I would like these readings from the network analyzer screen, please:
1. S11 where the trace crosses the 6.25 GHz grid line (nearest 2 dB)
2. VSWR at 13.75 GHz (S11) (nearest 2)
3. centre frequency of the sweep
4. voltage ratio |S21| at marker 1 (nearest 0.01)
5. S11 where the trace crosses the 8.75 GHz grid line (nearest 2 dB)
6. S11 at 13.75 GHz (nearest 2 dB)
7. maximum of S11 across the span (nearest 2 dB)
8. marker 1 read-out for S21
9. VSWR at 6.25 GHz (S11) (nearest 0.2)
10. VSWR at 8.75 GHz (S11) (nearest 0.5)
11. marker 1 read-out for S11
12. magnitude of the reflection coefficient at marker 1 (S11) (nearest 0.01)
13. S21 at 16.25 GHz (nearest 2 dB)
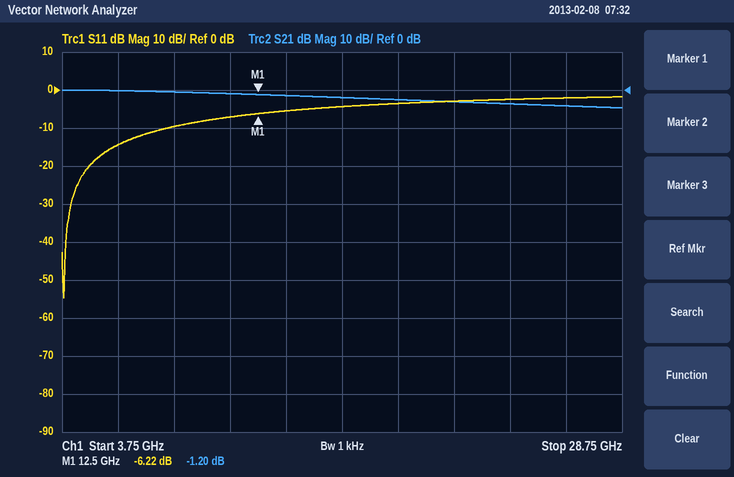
-14 dB
4
16.25 GHz
0.87
-10 dB
-6 dB
-2 dB
-1.20 dB
1.4
2.0
-6.22 dB
0.49
-2 dB
